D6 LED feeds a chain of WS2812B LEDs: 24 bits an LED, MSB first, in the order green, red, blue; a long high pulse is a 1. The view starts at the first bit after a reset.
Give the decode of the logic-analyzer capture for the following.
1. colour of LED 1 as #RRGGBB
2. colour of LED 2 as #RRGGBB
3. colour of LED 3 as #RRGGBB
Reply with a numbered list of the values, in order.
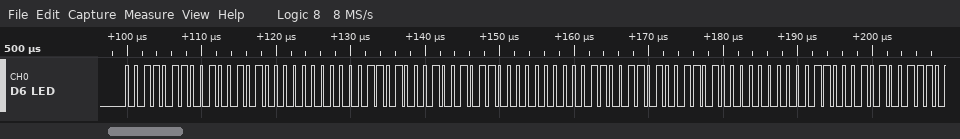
1. #4A3600
2. #4B3400
3. #4D3300
